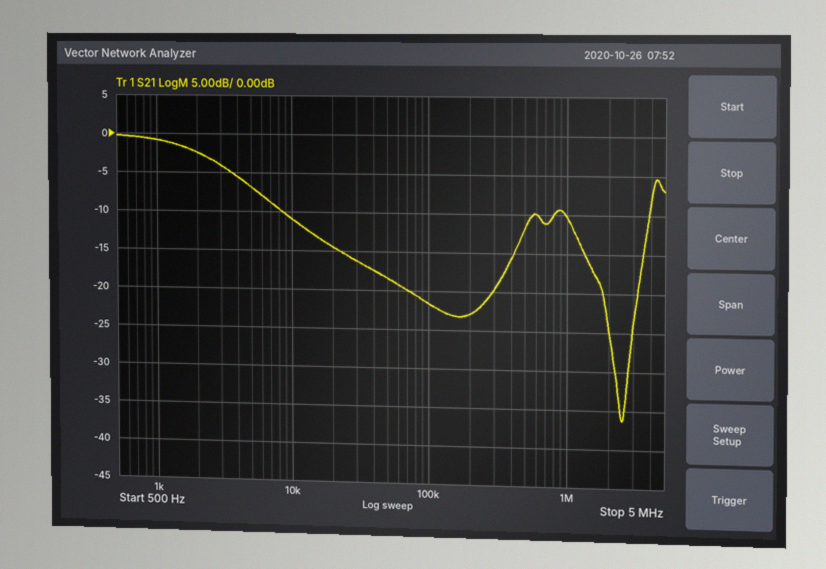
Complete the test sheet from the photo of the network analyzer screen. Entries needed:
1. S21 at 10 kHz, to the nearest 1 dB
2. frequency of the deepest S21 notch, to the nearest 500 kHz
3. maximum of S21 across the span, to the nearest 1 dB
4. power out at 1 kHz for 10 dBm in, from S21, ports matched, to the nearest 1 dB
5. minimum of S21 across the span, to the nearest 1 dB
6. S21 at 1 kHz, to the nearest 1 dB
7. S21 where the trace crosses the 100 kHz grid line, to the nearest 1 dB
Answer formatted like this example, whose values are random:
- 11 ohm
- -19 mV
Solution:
- -11 dB
- 2.5 MHz
- 0 dB
- 9 dBm
- -36 dB
- -1 dB
- -22 dB
